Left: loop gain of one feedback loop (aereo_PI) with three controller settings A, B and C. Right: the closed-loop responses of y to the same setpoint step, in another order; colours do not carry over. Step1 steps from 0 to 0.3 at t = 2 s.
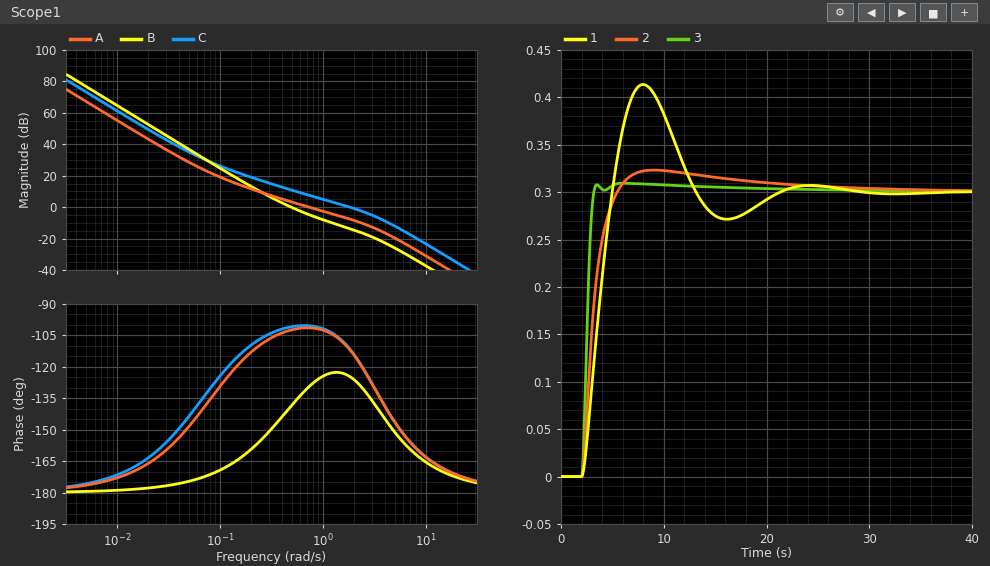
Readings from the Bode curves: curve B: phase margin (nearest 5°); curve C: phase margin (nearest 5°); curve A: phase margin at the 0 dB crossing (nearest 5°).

40°
70°
80°
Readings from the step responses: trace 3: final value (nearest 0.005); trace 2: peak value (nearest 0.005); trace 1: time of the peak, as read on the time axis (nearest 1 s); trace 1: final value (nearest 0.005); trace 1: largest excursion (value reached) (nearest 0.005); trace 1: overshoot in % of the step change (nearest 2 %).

0.300
0.325
8 s
0.300
0.415
38 %
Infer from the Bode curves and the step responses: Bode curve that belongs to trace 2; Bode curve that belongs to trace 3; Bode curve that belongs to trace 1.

A
C
B
